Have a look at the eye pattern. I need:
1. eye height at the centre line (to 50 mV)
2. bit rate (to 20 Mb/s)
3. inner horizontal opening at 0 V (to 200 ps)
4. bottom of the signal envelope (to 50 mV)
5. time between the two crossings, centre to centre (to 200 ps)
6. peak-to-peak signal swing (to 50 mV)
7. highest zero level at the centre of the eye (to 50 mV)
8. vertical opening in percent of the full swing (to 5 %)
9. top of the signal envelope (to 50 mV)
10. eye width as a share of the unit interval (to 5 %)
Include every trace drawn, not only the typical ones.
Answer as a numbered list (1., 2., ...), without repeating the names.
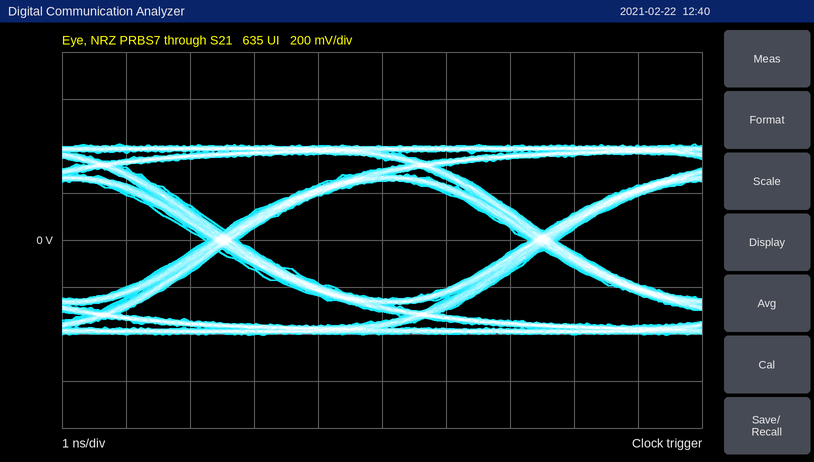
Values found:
1. 500 mV
2. 200 Mb/s
3. 4.6 ns
4. -400 mV
5. 5.0 ns
6. 800 mV
7. -250 mV
8. 60 %
9. 400 mV
10. 90 %
